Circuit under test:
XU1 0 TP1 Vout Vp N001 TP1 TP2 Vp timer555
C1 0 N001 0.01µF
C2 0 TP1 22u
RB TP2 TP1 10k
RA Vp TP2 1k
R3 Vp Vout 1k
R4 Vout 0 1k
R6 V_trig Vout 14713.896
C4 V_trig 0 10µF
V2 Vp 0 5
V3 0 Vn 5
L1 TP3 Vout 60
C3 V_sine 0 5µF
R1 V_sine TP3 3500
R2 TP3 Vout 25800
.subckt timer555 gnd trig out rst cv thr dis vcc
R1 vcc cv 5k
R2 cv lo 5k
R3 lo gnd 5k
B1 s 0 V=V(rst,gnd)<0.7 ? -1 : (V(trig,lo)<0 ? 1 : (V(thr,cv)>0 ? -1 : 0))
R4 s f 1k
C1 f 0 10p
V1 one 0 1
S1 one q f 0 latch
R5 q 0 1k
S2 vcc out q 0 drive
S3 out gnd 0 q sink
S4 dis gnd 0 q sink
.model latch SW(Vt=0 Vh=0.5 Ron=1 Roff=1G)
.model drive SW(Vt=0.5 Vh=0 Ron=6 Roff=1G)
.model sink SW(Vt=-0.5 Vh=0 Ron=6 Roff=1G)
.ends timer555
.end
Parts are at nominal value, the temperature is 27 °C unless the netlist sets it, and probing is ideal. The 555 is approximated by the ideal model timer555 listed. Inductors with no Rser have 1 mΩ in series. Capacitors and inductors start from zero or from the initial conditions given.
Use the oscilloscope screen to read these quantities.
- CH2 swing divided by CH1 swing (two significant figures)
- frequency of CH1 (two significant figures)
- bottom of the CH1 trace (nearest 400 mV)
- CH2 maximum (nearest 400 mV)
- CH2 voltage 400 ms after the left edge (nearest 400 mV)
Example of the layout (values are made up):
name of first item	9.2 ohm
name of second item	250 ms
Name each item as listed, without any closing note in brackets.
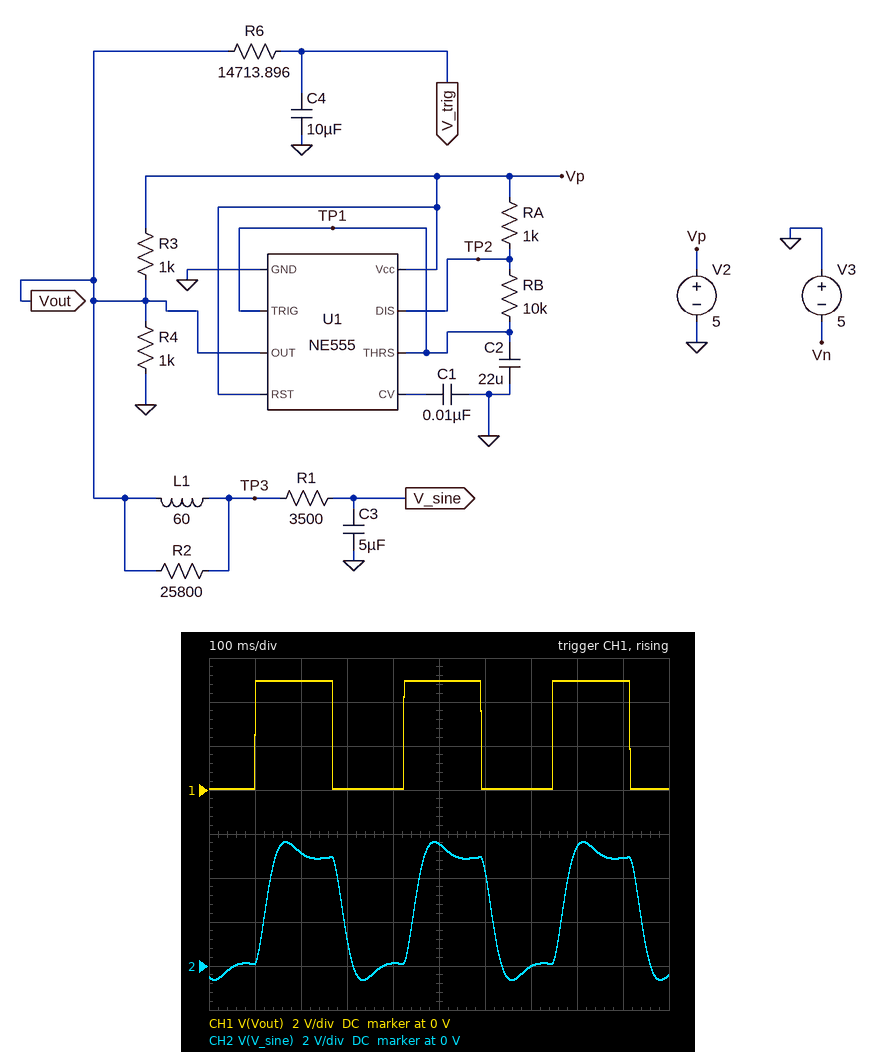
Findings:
CH2 swing divided by CH1 swing	1.3
frequency of CH1	3.1 Hz
bottom of the CH1 trace	0 V
CH2 maximum	5.6 V
CH2 voltage 400 ms after the left edge	0 V
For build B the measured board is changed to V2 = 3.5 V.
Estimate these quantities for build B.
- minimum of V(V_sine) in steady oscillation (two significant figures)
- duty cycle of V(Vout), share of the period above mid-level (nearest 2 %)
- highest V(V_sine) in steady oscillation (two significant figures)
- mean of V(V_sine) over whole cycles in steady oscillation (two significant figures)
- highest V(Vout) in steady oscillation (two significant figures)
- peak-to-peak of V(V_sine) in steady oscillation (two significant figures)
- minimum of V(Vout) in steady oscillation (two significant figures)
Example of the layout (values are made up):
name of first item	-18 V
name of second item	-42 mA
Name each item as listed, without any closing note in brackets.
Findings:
minimum of V(V_sine) in steady oscillation	-450 mV
duty cycle of V(Vout), share of the period above mid-level	52 %
highest V(V_sine) in steady oscillation	3.9 V
mean of V(V_sine) over whole cycles in steady oscillation	1.8 V
highest V(Vout) in steady oscillation	3.5 V
peak-to-peak of V(V_sine) in steady oscillation	4.4 V
minimum of V(Vout) in steady oscillation	21 mV
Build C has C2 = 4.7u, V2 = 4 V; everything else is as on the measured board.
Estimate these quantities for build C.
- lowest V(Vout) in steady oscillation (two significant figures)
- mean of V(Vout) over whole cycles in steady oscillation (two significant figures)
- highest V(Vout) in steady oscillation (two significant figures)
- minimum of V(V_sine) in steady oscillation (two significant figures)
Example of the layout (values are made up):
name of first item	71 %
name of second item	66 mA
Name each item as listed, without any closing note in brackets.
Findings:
lowest V(Vout) in steady oscillation	23 mV
mean of V(Vout) over whole cycles in steady oscillation	2.1 V
highest V(Vout) in steady oscillation	4.0 V
minimum of V(V_sine) in steady oscillation	1.1 V
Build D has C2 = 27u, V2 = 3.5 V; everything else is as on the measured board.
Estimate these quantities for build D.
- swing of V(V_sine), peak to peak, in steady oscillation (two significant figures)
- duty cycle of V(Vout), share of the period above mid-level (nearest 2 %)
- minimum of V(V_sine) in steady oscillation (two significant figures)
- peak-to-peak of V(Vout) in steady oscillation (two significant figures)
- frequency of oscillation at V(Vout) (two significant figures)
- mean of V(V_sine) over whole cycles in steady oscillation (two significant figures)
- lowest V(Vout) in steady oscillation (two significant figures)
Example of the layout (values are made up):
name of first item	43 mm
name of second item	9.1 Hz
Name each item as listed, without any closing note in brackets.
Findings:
swing of V(V_sine), peak to peak, in steady oscillation	4.4 V
duty cycle of V(Vout), share of the period above mid-level	52 %
minimum of V(V_sine) in steady oscillation	-450 mV
peak-to-peak of V(Vout) in steady oscillation	3.5 V
frequency of oscillation at V(Vout)	2.5 Hz
mean of V(V_sine) over whole cycles in steady oscillation	1.8 V
lowest V(Vout) in steady oscillation	21 mV
